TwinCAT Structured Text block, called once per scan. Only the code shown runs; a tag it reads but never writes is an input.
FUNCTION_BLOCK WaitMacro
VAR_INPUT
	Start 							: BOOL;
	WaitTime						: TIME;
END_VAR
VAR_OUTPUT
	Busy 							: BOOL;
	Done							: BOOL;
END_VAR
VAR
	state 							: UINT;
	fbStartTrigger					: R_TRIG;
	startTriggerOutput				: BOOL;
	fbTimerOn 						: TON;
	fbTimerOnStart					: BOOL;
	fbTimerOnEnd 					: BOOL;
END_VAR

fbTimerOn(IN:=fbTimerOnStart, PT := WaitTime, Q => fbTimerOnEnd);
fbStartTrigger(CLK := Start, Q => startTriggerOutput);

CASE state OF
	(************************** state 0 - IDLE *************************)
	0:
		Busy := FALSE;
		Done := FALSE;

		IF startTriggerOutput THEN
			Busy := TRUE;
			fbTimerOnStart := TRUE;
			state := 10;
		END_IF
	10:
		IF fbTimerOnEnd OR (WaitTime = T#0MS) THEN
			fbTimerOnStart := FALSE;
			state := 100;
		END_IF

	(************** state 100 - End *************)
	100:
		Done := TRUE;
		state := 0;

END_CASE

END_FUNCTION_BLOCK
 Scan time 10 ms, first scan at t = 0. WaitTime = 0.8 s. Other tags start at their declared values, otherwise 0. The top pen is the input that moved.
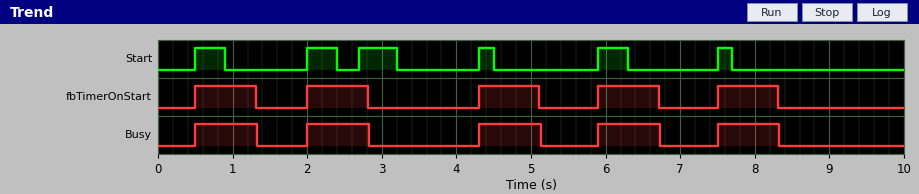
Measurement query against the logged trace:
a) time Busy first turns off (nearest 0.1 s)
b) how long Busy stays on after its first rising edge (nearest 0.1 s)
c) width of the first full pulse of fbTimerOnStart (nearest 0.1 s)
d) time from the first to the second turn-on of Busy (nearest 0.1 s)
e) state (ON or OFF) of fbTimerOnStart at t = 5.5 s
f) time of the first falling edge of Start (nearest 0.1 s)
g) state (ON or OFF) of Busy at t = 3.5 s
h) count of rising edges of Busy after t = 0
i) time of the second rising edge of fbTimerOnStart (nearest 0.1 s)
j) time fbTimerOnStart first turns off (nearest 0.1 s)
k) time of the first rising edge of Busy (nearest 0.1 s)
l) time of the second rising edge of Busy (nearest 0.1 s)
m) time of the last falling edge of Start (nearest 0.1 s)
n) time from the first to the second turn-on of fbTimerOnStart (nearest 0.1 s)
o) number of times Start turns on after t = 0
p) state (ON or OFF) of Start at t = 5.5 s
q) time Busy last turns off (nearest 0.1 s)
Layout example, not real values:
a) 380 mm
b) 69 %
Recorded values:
a) 1.3 s
b) 0.8 s
c) 0.8 s
d) 1.5 s
e) OFF
f) 0.9 s
g) OFF
h) 5
i) 2.0 s
j) 1.3 s
k) 0.5 s
l) 2.0 s
m) 7.7 s
n) 1.5 s
o) 6
p) OFF
q) 8.3 s
